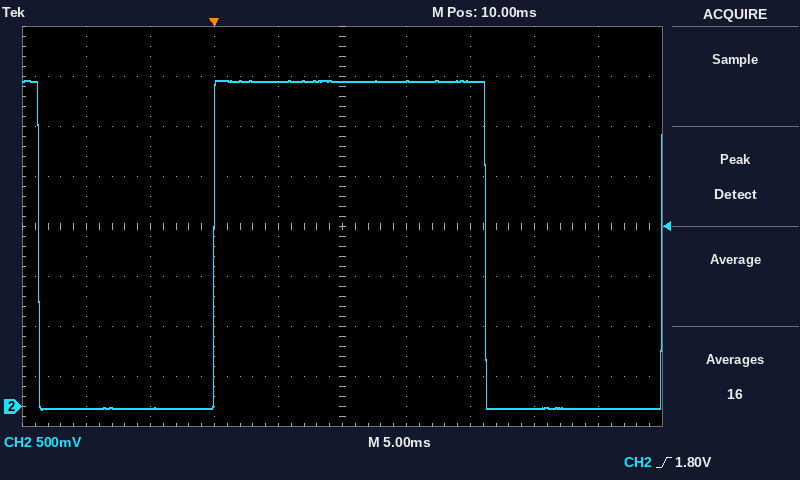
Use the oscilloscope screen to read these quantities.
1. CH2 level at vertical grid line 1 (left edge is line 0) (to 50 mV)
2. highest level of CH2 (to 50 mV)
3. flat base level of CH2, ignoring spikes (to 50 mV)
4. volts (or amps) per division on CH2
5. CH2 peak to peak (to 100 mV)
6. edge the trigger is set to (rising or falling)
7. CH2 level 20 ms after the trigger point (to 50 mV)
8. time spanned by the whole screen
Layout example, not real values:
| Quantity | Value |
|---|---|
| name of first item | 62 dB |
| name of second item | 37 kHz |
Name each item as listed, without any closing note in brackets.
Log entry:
| Quantity | Value |
|---|---|
| CH2 level at vertical grid line 1 (left edge is line 0) | 0 mV |
| highest level of CH2 | 3.25 V |
| flat base level of CH2, ignoring spikes | 0 mV |
| volts (or amps) per division on CH2 | 500 mV |
| CH2 peak to peak | 3.30 V |
| edge the trigger is set to | rising |
| CH2 level 20 ms after the trigger point | 3.25 V |
| time spanned by the whole screen | 50 ms |
